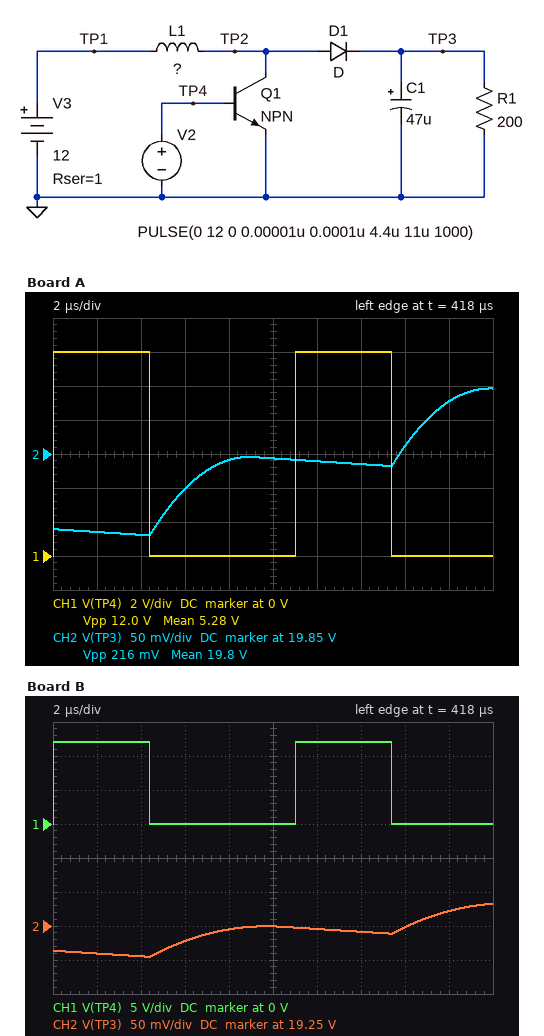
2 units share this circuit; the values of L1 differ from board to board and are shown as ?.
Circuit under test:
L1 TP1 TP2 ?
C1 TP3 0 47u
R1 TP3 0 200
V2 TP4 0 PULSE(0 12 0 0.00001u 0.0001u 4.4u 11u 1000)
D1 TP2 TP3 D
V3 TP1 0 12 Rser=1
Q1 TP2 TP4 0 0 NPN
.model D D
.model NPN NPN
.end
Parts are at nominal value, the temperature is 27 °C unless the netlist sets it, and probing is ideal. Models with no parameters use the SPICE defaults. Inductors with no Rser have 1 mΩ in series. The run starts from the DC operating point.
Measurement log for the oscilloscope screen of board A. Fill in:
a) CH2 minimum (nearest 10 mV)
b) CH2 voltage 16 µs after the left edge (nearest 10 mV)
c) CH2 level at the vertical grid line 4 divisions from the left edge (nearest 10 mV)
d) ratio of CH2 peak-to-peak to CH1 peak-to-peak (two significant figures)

19.73 V
19.86 V
19.84 V
0.018
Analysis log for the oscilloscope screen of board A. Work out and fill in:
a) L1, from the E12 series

18 µH
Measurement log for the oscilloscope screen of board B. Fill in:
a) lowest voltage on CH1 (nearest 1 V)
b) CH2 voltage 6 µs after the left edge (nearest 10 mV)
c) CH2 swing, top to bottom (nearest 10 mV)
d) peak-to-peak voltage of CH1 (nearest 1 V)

0 V
19.23 V
80 mV
12 V
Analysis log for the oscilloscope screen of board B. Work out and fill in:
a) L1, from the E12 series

56 µH
